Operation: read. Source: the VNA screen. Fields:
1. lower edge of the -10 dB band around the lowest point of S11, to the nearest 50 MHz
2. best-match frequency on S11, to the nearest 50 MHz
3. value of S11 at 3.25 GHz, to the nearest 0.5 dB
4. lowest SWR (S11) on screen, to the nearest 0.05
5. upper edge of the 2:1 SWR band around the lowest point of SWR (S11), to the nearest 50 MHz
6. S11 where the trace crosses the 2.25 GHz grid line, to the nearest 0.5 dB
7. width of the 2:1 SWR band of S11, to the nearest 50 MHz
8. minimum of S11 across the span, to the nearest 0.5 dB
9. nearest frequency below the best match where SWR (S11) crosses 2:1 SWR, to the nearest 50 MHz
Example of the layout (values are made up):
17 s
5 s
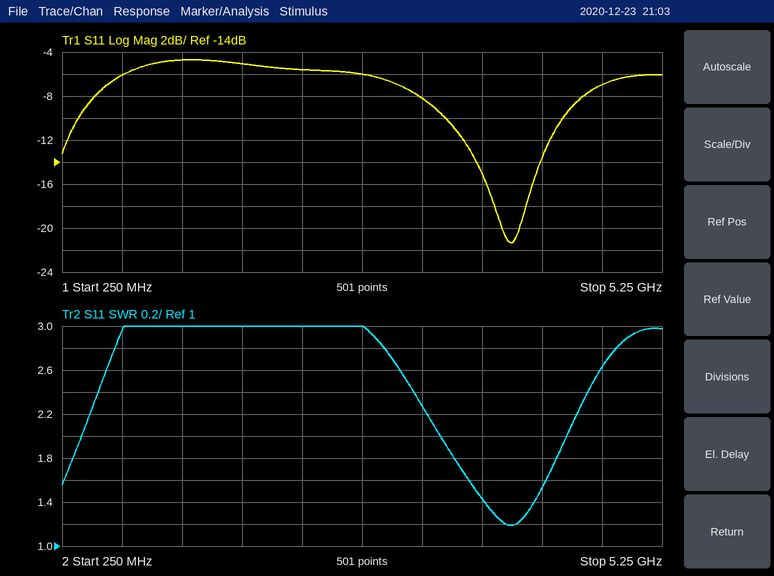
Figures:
3.45 GHz
4.00 GHz
-8.0 dB
1.20
4.45 GHz
-5.5 dB
1.05 GHz
-21.5 dB
3.40 GHz
